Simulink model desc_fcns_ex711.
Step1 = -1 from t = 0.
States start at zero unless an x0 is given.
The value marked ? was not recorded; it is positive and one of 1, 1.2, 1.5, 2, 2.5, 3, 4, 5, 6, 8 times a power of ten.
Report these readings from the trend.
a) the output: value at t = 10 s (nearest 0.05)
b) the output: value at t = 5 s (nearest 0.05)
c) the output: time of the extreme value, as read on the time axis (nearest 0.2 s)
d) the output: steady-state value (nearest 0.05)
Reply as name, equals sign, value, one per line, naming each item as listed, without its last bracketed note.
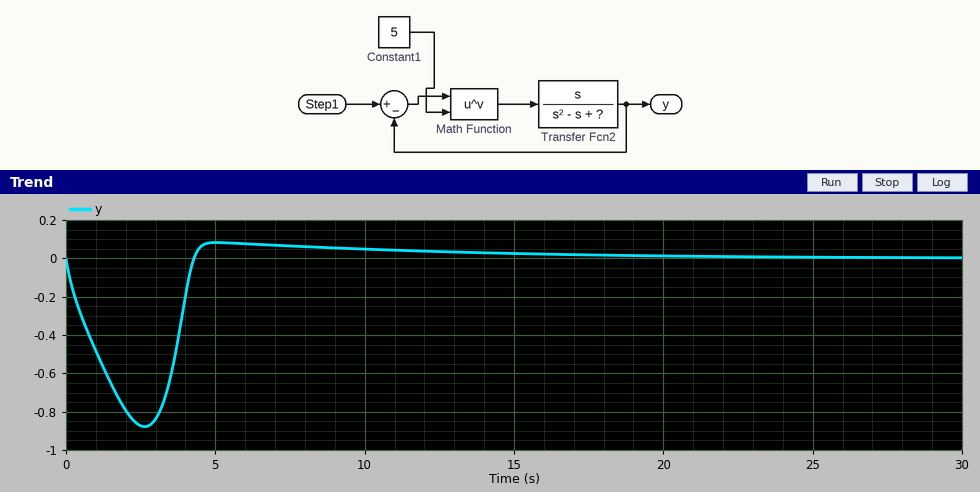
the output: value at t = 10 s = 0.05
the output: value at t = 5 s = 0.10
the output: time of the extreme value, as read on the time axis = 2.6 s
the output: steady-state value = 0.00
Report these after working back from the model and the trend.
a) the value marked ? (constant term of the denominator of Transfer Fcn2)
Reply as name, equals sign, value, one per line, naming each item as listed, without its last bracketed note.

the value marked ? = 0.6
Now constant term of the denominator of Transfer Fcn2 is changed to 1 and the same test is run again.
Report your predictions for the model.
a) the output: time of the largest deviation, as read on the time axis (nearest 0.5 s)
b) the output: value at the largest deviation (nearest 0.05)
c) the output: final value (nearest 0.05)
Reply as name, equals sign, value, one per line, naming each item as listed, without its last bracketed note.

the output: time of the largest deviation, as read on the time axis = 1.5 s
the output: value at the largest deviation = -0.50
the output: final value = 0.00
